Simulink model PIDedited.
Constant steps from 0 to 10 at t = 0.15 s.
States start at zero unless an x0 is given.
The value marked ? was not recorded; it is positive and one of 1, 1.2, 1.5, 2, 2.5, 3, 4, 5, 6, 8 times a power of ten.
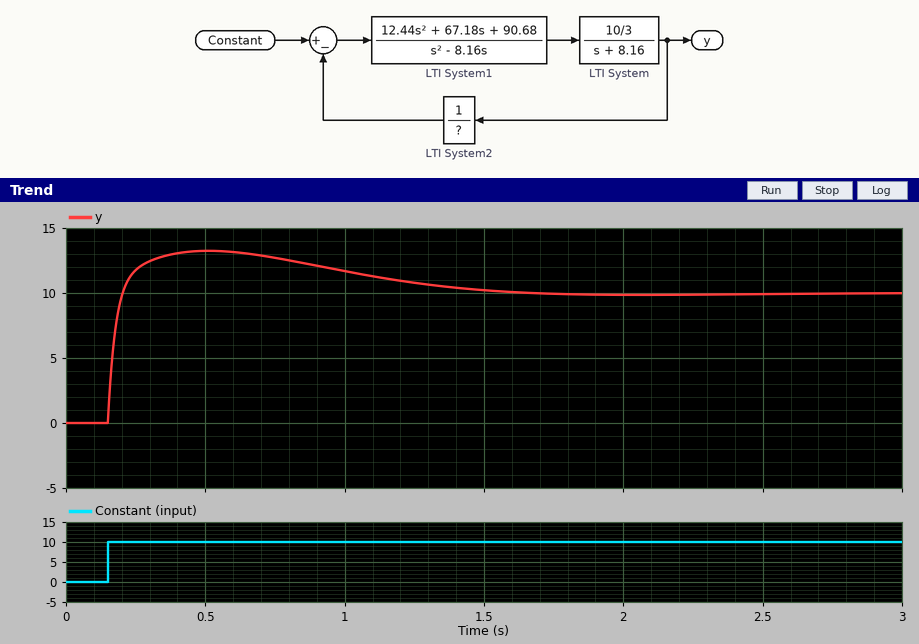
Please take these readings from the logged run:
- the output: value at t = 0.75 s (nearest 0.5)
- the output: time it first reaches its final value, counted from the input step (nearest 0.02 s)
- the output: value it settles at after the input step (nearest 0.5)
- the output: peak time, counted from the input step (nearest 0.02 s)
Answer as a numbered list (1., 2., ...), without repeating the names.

1. 12.5
2. 0.06 s
3. 10.0
4. 0.36 s
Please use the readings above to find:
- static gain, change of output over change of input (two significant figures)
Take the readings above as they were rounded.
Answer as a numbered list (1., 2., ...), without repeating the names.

1. 1.0
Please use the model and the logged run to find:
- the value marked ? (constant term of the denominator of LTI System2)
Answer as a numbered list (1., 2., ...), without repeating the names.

1. 1
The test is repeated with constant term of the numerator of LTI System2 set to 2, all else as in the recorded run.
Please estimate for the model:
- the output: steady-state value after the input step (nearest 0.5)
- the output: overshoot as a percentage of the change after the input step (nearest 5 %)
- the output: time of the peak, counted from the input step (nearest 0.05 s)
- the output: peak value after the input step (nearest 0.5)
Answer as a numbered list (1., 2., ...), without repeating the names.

1. 5.0
2. 15 %
3. 0.30 s
4. 5.5
